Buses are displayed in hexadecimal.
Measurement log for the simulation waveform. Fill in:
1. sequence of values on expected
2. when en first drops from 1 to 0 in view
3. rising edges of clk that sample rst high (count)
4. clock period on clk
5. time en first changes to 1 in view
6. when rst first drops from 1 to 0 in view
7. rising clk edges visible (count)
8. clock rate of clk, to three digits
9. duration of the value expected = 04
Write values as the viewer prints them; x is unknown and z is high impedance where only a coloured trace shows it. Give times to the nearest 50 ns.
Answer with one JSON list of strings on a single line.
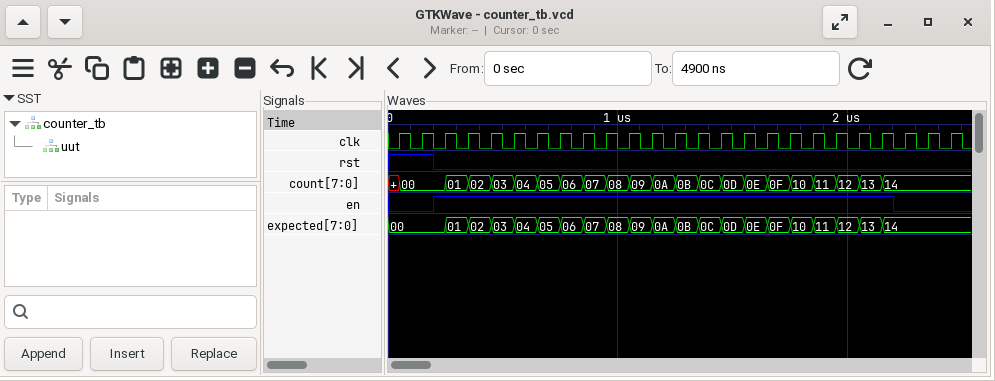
["00, 01, 02, 03, 04, 05, 06, 07, 08, 09, 0A, 0B, 0C, 0D, 0E, 0F, 10, 11, 12, 13, 14", "2200 ns", "2", "100 ns", "200 ns", "200 ns", "25", "10.0 MHz", "100 ns"]
